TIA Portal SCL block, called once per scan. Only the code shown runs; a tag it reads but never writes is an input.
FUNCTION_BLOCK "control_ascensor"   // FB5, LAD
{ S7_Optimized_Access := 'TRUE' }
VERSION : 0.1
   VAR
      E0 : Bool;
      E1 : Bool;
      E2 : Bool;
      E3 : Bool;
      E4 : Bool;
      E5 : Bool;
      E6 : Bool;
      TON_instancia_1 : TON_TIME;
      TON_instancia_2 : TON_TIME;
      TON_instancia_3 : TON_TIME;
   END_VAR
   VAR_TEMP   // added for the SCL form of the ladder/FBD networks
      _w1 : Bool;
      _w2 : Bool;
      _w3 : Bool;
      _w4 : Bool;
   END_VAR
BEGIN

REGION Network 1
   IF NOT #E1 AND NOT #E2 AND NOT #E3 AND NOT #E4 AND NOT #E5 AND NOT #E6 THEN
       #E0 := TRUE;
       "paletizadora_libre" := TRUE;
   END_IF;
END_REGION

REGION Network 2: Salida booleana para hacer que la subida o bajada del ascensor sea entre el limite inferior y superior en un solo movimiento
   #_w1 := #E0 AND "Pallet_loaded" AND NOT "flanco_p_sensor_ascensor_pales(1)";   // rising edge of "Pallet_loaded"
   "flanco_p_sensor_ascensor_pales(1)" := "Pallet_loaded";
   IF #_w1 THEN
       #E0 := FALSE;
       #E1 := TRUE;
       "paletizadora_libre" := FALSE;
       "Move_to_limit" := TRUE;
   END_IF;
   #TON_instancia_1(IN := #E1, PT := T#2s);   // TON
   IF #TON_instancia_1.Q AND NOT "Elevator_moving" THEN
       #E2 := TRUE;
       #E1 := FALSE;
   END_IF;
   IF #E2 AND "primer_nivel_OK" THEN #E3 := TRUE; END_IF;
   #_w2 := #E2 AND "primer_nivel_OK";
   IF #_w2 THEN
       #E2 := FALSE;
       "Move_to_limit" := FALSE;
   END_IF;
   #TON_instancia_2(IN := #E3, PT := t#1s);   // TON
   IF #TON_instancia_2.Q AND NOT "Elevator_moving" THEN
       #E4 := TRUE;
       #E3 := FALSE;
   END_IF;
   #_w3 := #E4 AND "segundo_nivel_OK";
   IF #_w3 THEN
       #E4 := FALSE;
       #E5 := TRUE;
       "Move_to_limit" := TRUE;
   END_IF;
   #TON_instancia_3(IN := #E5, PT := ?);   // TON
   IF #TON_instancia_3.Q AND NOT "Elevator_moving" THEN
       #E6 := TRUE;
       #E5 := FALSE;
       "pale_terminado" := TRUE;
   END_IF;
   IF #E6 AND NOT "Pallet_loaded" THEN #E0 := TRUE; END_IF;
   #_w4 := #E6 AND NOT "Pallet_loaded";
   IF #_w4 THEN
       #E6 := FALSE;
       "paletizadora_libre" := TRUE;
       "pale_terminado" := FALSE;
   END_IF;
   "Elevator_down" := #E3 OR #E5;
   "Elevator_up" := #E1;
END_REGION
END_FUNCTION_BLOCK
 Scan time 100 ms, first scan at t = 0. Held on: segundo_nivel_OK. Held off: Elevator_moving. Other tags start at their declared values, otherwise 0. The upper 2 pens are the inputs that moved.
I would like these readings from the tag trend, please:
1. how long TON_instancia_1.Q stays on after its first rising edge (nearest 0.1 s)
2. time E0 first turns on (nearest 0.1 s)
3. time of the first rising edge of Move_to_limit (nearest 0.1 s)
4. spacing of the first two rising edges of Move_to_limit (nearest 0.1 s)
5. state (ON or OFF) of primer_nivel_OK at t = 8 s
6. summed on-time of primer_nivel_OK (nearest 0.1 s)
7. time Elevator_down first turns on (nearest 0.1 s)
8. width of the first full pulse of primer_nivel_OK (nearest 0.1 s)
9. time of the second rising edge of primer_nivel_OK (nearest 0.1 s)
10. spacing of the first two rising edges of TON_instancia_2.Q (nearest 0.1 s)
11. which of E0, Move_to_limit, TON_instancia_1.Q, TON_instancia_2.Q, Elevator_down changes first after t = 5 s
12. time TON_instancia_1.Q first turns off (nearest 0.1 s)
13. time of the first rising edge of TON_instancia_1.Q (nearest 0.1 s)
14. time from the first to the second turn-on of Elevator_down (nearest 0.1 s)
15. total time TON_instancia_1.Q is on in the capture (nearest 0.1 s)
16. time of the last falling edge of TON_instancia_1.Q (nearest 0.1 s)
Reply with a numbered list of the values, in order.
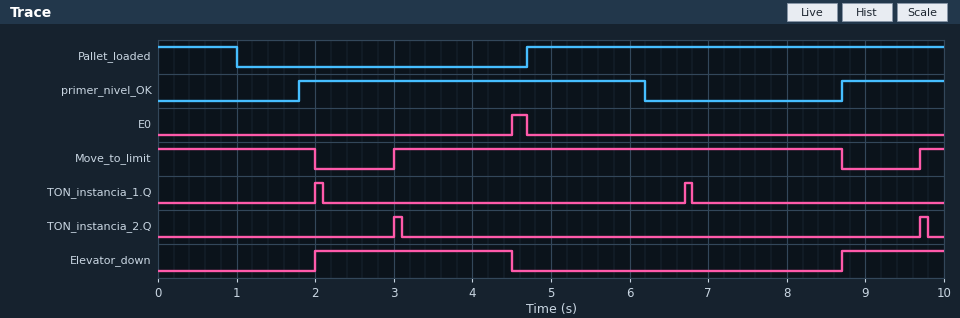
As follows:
1. 0.1 s
2. 4.5 s
3. 3.0 s
4. 6.7 s
5. OFF
6. 5.7 s
7. 2.0 s
8. 4.4 s
9. 8.7 s
10. 6.7 s
11. TON_instancia_1.Q
12. 2.1 s
13. 2.0 s
14. 6.7 s
15. 0.2 s
16. 6.8 s
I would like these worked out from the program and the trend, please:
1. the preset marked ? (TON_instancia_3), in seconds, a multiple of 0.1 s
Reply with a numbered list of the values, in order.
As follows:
1. 1.5 s
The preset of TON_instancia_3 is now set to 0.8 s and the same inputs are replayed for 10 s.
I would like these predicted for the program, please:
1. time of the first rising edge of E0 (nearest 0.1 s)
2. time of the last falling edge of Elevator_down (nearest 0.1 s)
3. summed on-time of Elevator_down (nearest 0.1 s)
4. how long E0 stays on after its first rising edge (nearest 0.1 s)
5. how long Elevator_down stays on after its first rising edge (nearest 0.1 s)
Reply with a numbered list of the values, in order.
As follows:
1. 3.8 s
2. 3.8 s
3. 3.1 s
4. 0.9 s
5. 1.8 s
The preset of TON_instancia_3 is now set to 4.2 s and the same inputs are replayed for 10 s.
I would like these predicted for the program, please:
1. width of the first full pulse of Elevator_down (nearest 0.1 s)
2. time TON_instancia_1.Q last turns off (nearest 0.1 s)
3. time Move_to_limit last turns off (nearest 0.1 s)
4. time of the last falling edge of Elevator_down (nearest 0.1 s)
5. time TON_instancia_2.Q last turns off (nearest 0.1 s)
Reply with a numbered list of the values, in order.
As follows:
1. 5.2 s
2. 2.1 s
3. 2.0 s
4. 7.2 s
5. 3.1 s
